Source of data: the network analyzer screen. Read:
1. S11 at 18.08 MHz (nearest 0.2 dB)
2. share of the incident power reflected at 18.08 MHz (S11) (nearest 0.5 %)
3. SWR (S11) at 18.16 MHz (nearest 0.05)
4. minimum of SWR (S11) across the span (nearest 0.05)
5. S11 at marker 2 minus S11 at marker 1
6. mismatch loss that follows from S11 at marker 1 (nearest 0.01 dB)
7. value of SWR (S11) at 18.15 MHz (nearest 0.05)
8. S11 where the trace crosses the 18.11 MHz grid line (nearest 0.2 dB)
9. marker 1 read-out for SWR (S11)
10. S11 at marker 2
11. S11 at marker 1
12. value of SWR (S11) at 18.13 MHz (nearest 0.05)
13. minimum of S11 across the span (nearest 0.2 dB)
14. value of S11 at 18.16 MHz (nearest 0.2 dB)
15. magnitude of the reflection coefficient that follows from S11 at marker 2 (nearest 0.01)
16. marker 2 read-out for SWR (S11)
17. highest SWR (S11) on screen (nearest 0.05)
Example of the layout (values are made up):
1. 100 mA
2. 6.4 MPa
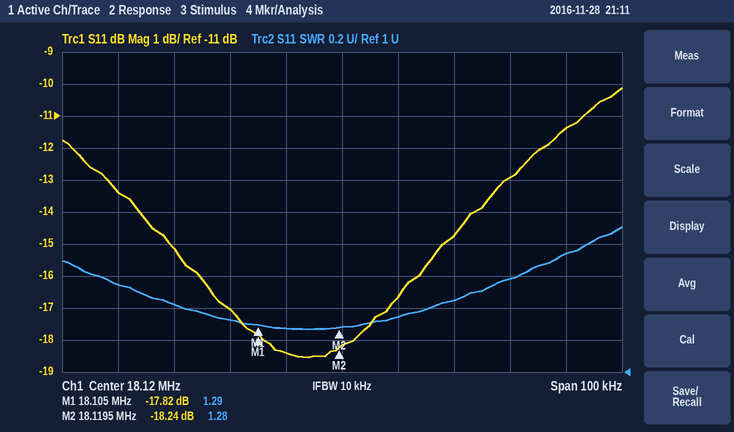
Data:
1. -13.4 dB
2. 4.5 %
3. 1.75
4. 1.25
5. -0.42 dB
6. 0.07 dB
7. 1.60
8. -18.4 dB
9. 1.29
10. -18.24 dB
11. -17.82 dB
12. 1.35
13. -18.6 dB
14. -11.4 dB
15. 0.12
16. 1.28
17. 1.90
